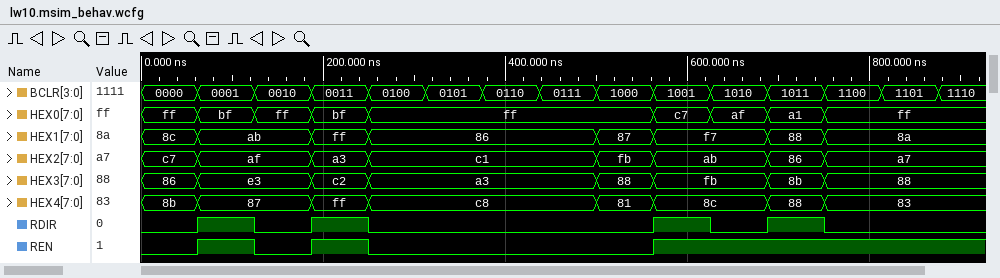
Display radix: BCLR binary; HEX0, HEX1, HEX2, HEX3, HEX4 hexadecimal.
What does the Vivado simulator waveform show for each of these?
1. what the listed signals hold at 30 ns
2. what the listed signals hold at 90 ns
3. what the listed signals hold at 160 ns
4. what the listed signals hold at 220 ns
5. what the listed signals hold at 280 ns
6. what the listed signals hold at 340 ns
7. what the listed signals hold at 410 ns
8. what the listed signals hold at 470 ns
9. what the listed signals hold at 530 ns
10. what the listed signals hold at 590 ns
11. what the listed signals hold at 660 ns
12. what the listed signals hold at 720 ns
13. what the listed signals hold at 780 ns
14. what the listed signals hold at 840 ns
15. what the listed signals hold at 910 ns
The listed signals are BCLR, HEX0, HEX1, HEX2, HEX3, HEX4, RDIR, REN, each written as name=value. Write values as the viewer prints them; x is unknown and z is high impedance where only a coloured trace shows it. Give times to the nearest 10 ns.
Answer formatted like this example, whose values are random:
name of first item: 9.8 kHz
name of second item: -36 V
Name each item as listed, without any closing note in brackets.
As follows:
what the listed signals hold at 30 ns: BCLR=0000, HEX0=ff, HEX1=8c, HEX2=c7, HEX3=86, HEX4=8b, RDIR=0, REN=0
what the listed signals hold at 90 ns: BCLR=0001, HEX0=bf, HEX1=ab, HEX2=af, HEX3=e3, HEX4=87, RDIR=1, REN=1
what the listed signals hold at 160 ns: BCLR=0010, HEX0=ff, HEX1=ab, HEX2=af, HEX3=e3, HEX4=87, RDIR=0, REN=0
what the listed signals hold at 220 ns: BCLR=0011, HEX0=bf, HEX1=ff, HEX2=a3, HEX3=c2, HEX4=ff, RDIR=1, REN=1
what the listed signals hold at 280 ns: BCLR=0100, HEX0=ff, HEX1=86, HEX2=c1, HEX3=a3, HEX4=c8, RDIR=0, REN=0
what the listed signals hold at 340 ns: BCLR=0101, HEX0=ff, HEX1=86, HEX2=c1, HEX3=a3, HEX4=c8, RDIR=0, REN=0
what the listed signals hold at 410 ns: BCLR=0110, HEX0=ff, HEX1=86, HEX2=c1, HEX3=a3, HEX4=c8, RDIR=0, REN=0
what the listed signals hold at 470 ns: BCLR=0111, HEX0=ff, HEX1=86, HEX2=c1, HEX3=a3, HEX4=c8, RDIR=0, REN=0
what the listed signals hold at 530 ns: BCLR=1000, HEX0=ff, HEX1=87, HEX2=fb, HEX3=88, HEX4=81, RDIR=0, REN=0
what the listed signals hold at 590 ns: BCLR=1001, HEX0=c7, HEX1=f7, HEX2=ab, HEX3=fb, HEX4=8c, RDIR=1, REN=1
what the listed signals hold at 660 ns: BCLR=1010, HEX0=af, HEX1=f7, HEX2=ab, HEX3=fb, HEX4=8c, RDIR=0, REN=1
what the listed signals hold at 720 ns: BCLR=1011, HEX0=a1, HEX1=88, HEX2=86, HEX3=8b, HEX4=88, RDIR=1, REN=1
what the listed signals hold at 780 ns: BCLR=1100, HEX0=ff, HEX1=8a, HEX2=a7, HEX3=88, HEX4=83, RDIR=0, REN=1
what the listed signals hold at 840 ns: BCLR=1101, HEX0=ff, HEX1=8a, HEX2=a7, HEX3=88, HEX4=83, RDIR=0, REN=1
what the listed signals hold at 910 ns: BCLR=1110, HEX0=ff, HEX1=8a, HEX2=a7, HEX3=88, HEX4=83, RDIR=0, REN=1
